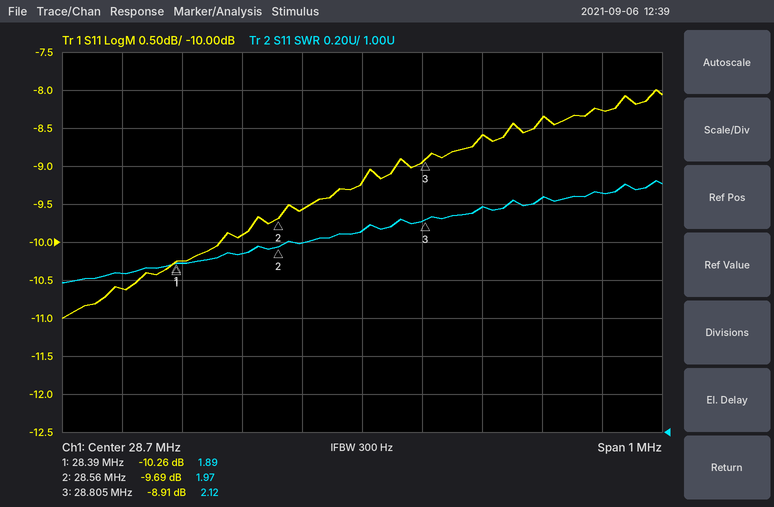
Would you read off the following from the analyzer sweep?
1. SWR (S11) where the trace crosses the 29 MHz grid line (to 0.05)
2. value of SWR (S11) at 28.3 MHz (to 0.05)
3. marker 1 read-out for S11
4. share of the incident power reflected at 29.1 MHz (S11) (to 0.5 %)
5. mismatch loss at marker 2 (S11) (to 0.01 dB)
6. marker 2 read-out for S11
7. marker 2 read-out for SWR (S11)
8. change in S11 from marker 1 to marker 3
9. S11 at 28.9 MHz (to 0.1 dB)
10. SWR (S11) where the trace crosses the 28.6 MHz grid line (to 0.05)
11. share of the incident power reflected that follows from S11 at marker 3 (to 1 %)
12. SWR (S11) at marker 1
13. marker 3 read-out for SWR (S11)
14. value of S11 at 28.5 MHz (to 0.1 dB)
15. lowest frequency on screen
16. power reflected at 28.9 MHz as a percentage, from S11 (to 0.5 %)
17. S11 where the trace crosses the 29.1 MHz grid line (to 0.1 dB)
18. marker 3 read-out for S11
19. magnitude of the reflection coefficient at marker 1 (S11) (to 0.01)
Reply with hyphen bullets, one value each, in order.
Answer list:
- 2.25
- 1.85
- -10.26 dB
- 15.0 %
- 0.49 dB
- -9.69 dB
- 1.97
- 1.35 dB
- -8.6 dB
- 2.00
- 13 %
- 1.89
- 2.12
- -9.9 dB
- 28.2 MHz
- 14.0 %
- -8.3 dB
- -8.91 dB
- 0.31
